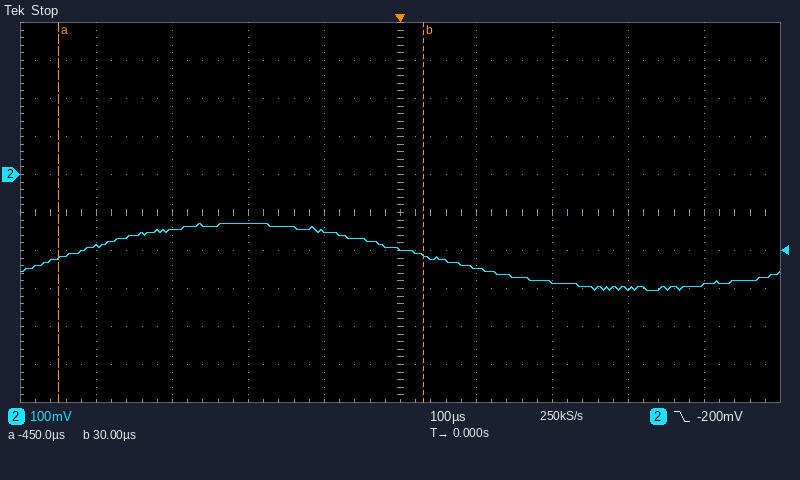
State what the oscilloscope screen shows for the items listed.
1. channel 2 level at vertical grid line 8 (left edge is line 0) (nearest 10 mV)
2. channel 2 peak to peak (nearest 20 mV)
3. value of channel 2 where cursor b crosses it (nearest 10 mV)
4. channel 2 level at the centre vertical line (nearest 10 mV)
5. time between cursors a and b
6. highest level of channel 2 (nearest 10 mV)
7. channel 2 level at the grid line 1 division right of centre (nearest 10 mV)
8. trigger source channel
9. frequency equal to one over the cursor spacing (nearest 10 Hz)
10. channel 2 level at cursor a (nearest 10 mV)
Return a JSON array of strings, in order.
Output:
["-300 mV", "180 mV", "-210 mV", "-200 mV", "480 µs", "-130 mV", "-250 mV", "channel 2", "2.08 kHz", "-220 mV"]
